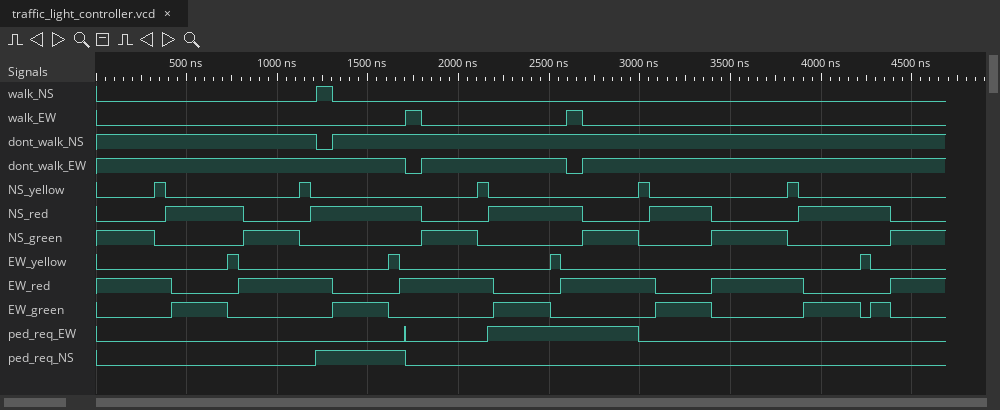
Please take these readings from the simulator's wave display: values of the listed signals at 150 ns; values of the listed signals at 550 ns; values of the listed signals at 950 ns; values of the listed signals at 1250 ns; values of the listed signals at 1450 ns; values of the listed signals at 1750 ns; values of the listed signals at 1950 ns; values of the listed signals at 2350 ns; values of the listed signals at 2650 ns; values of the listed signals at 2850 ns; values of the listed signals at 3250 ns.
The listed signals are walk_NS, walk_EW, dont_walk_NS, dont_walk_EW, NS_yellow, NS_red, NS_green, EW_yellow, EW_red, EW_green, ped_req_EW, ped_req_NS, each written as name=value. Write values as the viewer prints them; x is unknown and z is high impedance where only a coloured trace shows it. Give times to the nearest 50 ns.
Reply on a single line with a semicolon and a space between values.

walk_NS=0, walk_EW=0, dont_walk_NS=1, dont_walk_EW=1, NS_yellow=0, NS_red=0, NS_green=1, EW_yellow=0, EW_red=1, EW_green=0, ped_req_EW=0, ped_req_NS=0; walk_NS=0, walk_EW=0, dont_walk_NS=1, dont_walk_EW=1, NS_yellow=0, NS_red=1, NS_green=0, EW_yellow=0, EW_red=0, EW_green=1, ped_req_EW=0, ped_req_NS=0; walk_NS=0, walk_EW=0, dont_walk_NS=1, dont_walk_EW=1, NS_yellow=0, NS_red=0, NS_green=1, EW_yellow=0, EW_red=1, EW_green=0, ped_req_EW=0, ped_req_NS=0; walk_NS=1, walk_EW=0, dont_walk_NS=0, dont_walk_EW=1, NS_yellow=0, NS_red=1, NS_green=0, EW_yellow=0, EW_red=1, EW_green=0, ped_req_EW=0, ped_req_NS=1; walk_NS=0, walk_EW=0, dont_walk_NS=1, dont_walk_EW=1, NS_yellow=0, NS_red=1, NS_green=0, EW_yellow=0, EW_red=0, EW_green=1, ped_req_EW=0, ped_req_NS=1; walk_NS=0, walk_EW=1, dont_walk_NS=1, dont_walk_EW=0, NS_yellow=0, NS_red=1, NS_green=0, EW_yellow=0, EW_red=1, EW_green=0, ped_req_EW=0, ped_req_NS=0; walk_NS=0, walk_EW=0, dont_walk_NS=1, dont_walk_EW=1, NS_yellow=0, NS_red=0, NS_green=1, EW_yellow=0, EW_red=1, EW_green=0, ped_req_EW=0, ped_req_NS=0; walk_NS=0, walk_EW=0, dont_walk_NS=1, dont_walk_EW=1, NS_yellow=0, NS_red=1, NS_green=0, EW_yellow=0, EW_red=0, EW_green=1, ped_req_EW=1, ped_req_NS=0; walk_NS=0, walk_EW=1, dont_walk_NS=1, dont_walk_EW=0, NS_yellow=0, NS_red=1, NS_green=0, EW_yellow=0, EW_red=1, EW_green=0, ped_req_EW=1, ped_req_NS=0; walk_NS=0, walk_EW=0, dont_walk_NS=1, dont_walk_EW=1, NS_yellow=0, NS_red=0, NS_green=1, EW_yellow=0, EW_red=1, EW_green=0, ped_req_EW=1, ped_req_NS=0; walk_NS=0, walk_EW=0, dont_walk_NS=1, dont_walk_EW=1, NS_yellow=0, NS_red=1, NS_green=0, EW_yellow=0, EW_red=0, EW_green=1, ped_req_EW=0, ped_req_NS=0
